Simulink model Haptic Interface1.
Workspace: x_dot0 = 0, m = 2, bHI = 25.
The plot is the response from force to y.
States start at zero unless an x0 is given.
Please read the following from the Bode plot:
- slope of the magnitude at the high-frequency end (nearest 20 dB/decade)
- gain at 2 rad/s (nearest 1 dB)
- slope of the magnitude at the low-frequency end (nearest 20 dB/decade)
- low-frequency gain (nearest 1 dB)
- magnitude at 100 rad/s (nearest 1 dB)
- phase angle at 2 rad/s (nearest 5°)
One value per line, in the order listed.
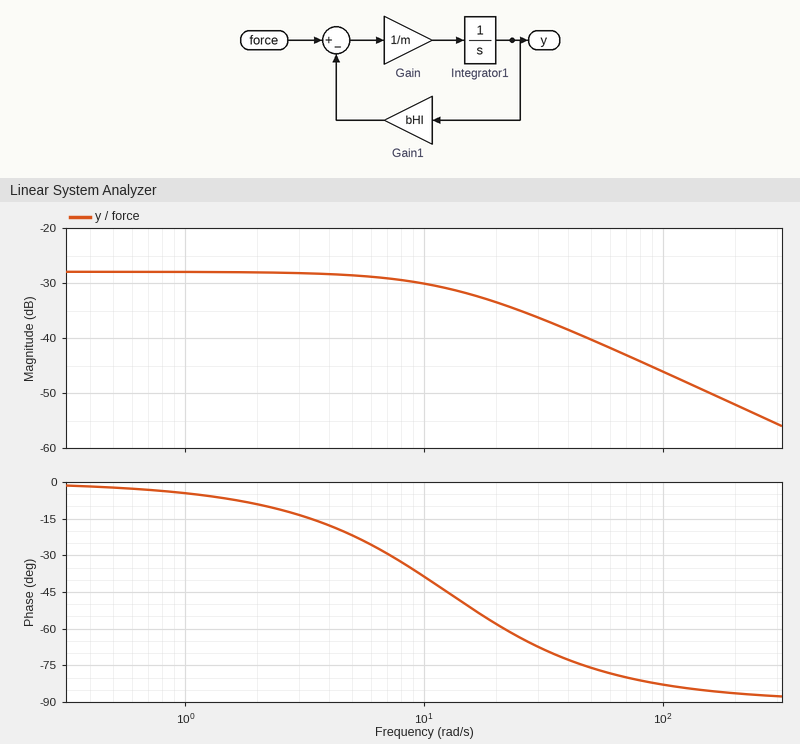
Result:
-20 dB/decade
-28 dB
0 dB/decade
-28 dB
-46 dB
-10°
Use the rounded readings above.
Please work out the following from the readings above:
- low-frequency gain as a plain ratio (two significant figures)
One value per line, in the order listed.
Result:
0.040
